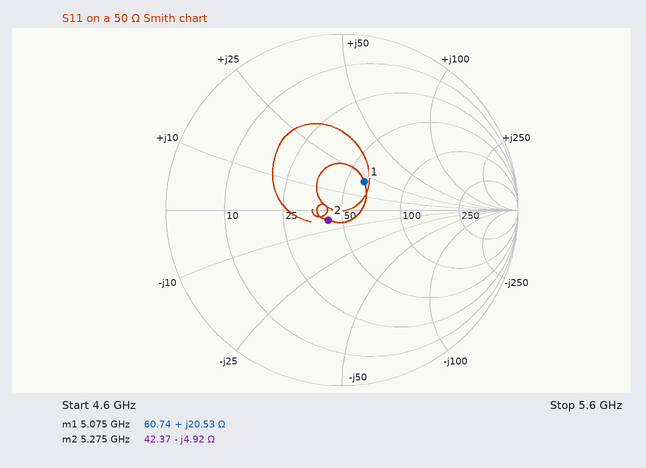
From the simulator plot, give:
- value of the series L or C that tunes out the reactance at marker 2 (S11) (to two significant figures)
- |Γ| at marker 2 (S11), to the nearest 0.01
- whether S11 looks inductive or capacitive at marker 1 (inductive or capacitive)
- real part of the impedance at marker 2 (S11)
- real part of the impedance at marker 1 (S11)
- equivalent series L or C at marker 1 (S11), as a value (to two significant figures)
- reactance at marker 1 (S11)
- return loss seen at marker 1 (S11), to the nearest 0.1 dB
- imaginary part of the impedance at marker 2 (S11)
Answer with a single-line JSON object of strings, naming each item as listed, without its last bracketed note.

{"value of the series L or C that tunes out the reactance at marker 2 (S11)": "150 pH", "|Γ| at marker 2 (S11), to the nearest 0.01": "0.10", "whether S11 looks inductive or capacitive at marker 1": "inductive", "real part of the impedance at marker 2": "42.37 Ω", "real part of the impedance at marker 1": "60.74 Ω", "equivalent series L or C at marker 1 (S11), as a value": "640 pH", "reactance at marker 1": "+20.53 Ω", "return loss seen at marker 1 (S11), to the nearest 0.1 dB": "13.7 dB", "imaginary part of the impedance at marker 2": "-4.92 Ω"}
